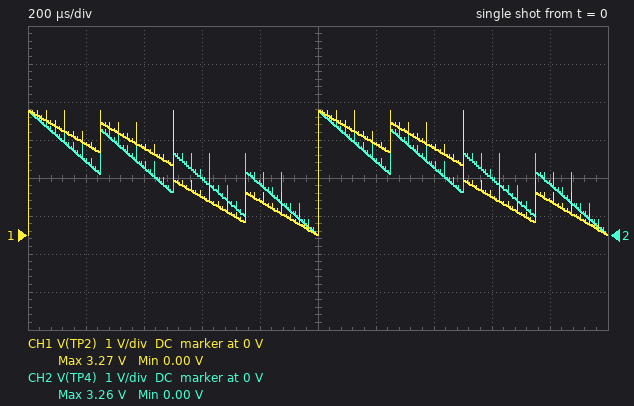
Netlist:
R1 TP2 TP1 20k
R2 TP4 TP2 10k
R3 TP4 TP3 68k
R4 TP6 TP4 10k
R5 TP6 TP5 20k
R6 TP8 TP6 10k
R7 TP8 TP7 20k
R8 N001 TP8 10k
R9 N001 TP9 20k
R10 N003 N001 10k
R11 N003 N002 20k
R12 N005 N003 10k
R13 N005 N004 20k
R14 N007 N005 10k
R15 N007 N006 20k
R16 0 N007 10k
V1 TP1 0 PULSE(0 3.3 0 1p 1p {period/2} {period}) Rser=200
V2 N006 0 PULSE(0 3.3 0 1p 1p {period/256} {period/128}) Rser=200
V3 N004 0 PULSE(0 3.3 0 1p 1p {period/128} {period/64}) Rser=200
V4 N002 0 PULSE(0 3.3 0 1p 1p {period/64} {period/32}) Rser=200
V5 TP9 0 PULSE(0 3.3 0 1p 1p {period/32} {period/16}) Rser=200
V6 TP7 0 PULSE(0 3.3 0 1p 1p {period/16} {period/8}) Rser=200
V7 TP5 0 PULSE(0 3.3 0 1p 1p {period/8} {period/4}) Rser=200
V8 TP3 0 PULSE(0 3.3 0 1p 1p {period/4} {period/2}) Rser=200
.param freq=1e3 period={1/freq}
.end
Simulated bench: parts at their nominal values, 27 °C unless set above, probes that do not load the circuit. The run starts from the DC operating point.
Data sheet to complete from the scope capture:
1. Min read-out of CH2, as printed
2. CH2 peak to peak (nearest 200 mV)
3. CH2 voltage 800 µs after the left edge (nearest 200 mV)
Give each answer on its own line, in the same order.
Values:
0.00 V
3.2 V
1.4 V
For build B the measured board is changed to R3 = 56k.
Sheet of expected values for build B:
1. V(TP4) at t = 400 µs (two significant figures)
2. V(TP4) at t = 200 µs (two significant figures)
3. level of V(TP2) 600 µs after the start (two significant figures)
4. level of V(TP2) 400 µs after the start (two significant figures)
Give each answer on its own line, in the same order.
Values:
1.7 V
2.0 V
1.0 V
2.2 V
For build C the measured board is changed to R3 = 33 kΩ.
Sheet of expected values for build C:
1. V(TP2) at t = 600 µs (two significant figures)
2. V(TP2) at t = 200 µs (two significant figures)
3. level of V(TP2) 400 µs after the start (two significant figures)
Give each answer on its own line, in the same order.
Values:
1.2 V
2.5 V
2.1 V
